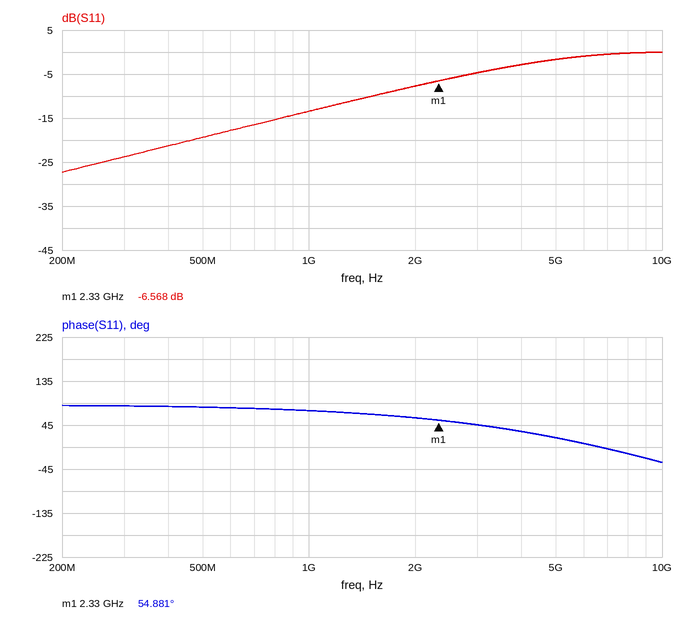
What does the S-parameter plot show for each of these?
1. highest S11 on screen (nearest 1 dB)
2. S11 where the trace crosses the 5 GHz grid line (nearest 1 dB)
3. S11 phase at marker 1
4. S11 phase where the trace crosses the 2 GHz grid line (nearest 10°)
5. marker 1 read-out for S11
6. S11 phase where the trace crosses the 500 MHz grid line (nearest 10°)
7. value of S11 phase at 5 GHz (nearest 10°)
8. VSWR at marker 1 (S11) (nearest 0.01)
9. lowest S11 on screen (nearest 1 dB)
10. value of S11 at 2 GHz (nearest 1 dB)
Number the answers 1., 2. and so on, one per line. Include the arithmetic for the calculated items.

1. 0 dB
2. -2 dB
3. 54.881°
4. 60°
5. -6.568 dB
6. 80°
7. 20°
8. (1 + 0.4695)/(1 − 0.4695) ≈ 2.77
9. -27 dB
10. -8 dB
